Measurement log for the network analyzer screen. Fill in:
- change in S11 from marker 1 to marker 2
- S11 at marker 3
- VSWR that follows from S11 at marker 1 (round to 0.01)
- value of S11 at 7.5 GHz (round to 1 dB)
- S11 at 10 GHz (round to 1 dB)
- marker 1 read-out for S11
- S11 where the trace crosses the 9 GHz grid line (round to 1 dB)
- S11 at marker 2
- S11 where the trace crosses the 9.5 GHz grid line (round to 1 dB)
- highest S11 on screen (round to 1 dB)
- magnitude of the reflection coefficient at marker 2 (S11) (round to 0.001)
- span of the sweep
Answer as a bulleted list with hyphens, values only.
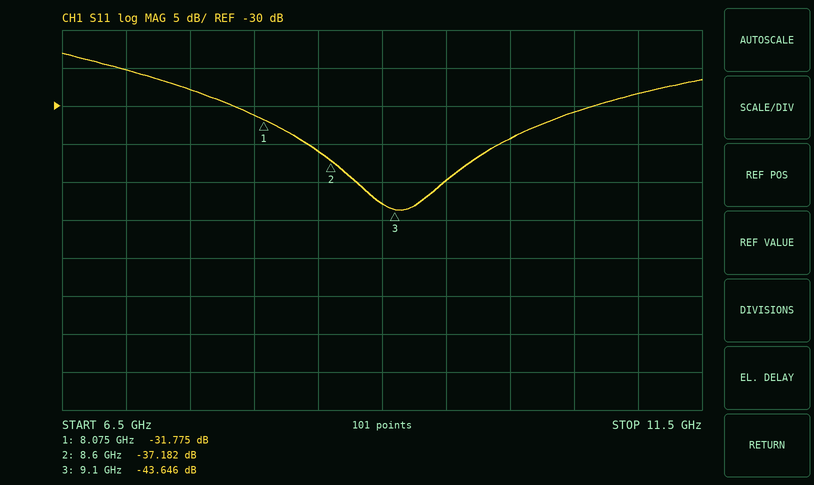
- -5.407 dB
- -43.646 dB
- 1.05
- -28 dB
- -34 dB
- -31.775 dB
- -43 dB
- -37.182 dB
- -40 dB
- -23 dB
- 0.014
- 5 GHz
